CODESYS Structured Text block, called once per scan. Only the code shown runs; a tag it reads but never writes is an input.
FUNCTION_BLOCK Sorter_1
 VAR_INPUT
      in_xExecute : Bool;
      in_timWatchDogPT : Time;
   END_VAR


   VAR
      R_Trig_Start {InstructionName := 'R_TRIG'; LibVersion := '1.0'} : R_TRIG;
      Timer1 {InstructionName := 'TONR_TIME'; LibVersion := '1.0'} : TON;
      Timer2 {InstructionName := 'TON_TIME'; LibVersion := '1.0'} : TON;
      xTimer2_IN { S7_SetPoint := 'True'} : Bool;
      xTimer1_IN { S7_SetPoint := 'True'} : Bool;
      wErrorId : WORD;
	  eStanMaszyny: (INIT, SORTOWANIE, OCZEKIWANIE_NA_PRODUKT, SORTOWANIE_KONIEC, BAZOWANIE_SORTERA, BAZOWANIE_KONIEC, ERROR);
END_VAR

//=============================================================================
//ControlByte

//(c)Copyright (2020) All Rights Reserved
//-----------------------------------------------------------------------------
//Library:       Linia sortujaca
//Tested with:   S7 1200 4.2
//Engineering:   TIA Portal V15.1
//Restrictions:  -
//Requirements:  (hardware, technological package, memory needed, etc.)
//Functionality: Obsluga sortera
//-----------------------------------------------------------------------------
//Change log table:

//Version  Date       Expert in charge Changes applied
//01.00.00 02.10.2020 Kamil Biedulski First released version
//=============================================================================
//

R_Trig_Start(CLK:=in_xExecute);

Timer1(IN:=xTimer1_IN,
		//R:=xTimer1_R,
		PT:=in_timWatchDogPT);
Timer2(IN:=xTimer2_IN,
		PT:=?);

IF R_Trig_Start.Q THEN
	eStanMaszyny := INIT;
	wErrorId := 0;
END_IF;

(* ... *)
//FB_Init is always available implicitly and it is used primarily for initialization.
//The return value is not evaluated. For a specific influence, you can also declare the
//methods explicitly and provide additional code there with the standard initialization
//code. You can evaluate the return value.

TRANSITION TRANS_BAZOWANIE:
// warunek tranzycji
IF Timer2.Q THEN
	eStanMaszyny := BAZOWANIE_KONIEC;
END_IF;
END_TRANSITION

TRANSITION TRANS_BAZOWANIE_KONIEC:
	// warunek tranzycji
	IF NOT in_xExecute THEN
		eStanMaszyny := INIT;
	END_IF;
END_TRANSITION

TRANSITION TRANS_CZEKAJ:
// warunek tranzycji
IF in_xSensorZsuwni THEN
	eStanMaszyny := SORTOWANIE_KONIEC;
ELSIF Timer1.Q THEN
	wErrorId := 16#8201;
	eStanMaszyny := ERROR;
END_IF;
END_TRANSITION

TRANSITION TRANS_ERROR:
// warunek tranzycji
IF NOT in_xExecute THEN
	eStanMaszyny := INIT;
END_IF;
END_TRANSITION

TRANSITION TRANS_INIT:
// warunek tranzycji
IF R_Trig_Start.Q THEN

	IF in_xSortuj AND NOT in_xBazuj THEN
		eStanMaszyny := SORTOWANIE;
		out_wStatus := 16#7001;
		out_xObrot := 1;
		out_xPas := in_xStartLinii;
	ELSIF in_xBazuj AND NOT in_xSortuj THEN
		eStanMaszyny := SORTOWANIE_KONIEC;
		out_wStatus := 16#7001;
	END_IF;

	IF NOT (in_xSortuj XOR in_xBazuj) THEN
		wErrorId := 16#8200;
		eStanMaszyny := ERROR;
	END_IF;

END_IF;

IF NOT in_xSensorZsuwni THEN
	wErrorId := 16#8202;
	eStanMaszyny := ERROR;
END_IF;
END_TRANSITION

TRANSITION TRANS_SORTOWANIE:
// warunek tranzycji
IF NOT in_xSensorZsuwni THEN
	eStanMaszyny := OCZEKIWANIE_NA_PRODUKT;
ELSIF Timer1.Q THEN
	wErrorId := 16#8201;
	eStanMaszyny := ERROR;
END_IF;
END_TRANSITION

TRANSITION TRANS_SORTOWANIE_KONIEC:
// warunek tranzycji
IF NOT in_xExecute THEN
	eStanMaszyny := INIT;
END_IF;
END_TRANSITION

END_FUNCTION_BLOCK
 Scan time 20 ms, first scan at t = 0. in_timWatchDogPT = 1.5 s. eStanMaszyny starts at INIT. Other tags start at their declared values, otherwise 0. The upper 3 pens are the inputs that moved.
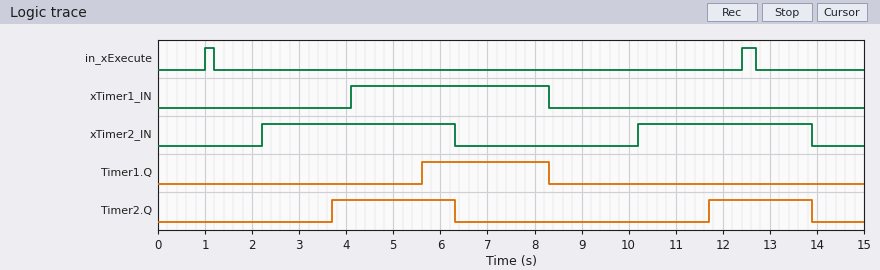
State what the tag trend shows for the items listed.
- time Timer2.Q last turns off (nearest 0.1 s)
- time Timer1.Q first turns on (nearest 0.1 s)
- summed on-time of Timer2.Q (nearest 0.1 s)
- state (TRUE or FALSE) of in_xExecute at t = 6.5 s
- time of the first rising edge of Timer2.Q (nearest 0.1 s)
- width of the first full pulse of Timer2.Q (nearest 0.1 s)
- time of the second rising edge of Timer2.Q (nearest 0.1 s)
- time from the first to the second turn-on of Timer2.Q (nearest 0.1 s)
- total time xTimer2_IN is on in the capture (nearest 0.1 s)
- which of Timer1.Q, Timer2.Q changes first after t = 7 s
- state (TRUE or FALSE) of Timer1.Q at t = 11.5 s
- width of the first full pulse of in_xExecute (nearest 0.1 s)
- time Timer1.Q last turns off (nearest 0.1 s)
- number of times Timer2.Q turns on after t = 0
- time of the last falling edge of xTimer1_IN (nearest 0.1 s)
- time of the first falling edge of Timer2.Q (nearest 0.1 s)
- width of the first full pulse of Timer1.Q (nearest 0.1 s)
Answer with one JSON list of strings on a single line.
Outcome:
["13.9 s", "5.6 s", "4.8 s", "FALSE", "3.7 s", "2.6 s", "11.7 s", "8.0 s", "7.8 s", "Timer1.Q", "FALSE", "0.2 s", "8.3 s", "2", "8.3 s", "6.3 s", "2.7 s"]
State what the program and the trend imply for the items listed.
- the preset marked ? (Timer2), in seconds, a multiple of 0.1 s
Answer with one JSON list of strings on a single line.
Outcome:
["1.5 s"]
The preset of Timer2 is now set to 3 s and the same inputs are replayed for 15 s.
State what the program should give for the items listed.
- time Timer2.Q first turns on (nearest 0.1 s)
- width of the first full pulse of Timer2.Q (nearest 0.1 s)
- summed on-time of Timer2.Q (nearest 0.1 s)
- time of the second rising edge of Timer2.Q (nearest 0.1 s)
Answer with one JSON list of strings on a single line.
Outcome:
["5.2 s", "1.1 s", "1.8 s", "13.2 s"]
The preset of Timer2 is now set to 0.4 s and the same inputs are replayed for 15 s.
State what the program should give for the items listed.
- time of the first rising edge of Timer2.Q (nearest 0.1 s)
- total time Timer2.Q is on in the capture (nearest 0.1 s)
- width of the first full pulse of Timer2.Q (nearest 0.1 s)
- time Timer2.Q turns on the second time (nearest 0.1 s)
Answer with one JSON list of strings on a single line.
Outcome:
["2.6 s", "7.0 s", "3.7 s", "10.6 s"]
